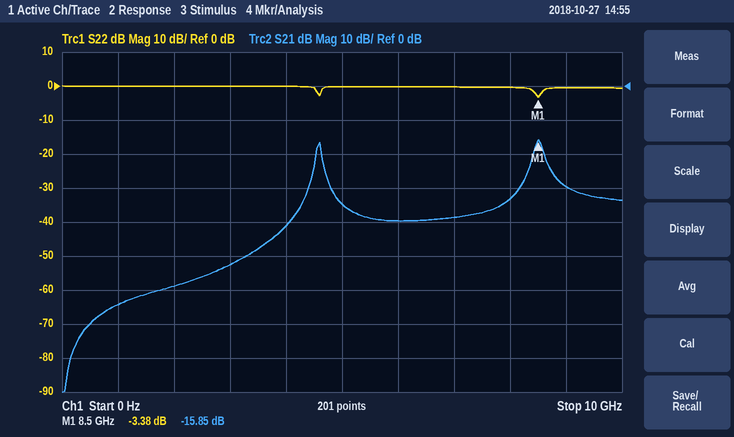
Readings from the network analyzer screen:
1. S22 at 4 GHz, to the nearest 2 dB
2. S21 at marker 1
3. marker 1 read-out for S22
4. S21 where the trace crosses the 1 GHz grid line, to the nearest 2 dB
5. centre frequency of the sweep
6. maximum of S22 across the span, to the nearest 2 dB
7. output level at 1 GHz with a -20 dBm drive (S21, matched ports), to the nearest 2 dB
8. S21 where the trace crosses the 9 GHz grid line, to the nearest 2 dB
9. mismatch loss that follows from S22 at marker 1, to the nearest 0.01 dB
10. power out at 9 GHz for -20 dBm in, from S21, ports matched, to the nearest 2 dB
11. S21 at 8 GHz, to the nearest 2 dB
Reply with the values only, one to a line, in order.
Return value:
0 dB
-15.85 dB
-3.38 dB
-64 dB
5 GHz
0 dB
-84 dBm
-30 dB
2.67 dB
-50 dBm
-34 dB
